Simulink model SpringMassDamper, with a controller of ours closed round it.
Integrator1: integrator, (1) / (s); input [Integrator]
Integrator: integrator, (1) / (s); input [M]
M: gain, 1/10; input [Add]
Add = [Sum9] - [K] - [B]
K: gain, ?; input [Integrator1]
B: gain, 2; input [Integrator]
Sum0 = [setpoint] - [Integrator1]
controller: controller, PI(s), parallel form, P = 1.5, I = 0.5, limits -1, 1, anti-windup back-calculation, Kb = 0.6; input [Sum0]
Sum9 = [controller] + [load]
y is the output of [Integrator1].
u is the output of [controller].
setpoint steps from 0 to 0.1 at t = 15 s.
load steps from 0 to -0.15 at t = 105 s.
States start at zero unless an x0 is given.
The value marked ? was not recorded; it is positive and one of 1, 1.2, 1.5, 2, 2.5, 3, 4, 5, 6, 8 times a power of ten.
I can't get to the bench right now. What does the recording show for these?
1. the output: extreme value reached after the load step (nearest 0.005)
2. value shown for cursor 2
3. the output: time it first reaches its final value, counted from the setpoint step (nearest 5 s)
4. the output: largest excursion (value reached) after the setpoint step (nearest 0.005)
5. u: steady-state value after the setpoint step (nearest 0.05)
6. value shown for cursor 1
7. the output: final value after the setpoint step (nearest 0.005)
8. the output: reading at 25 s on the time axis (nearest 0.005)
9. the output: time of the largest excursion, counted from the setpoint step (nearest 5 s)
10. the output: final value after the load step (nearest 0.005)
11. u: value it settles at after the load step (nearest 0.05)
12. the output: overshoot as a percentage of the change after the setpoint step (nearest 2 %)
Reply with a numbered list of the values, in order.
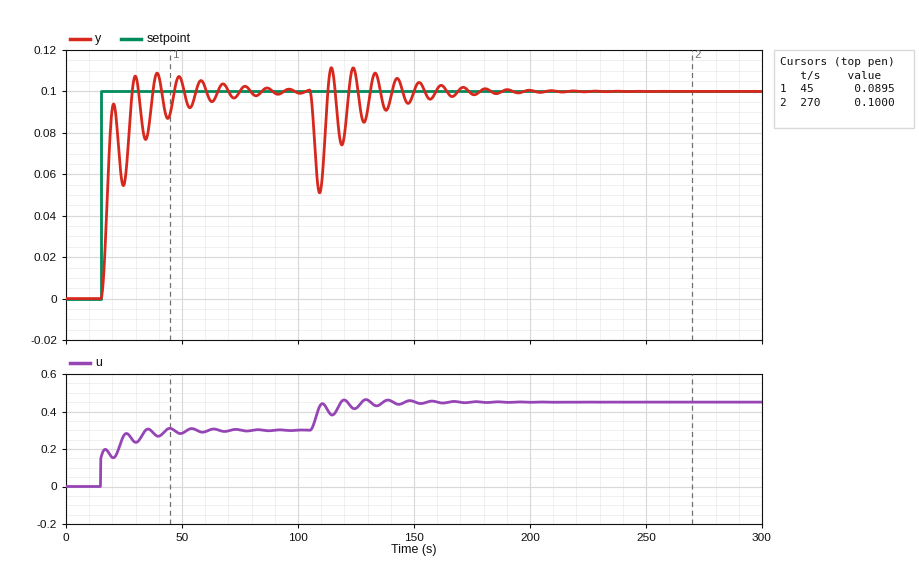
1. 0.050
2. 0.1000
3. 15 s
4. 0.110
5. 0.30
6. 0.0895
7. 0.100
8. 0.055
9. 25 s
10. 0.100
11. 0.45
12. 8 %
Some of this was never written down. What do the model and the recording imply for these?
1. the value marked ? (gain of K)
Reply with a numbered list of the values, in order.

1. 3
